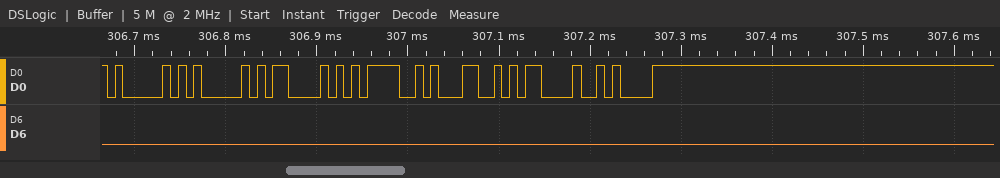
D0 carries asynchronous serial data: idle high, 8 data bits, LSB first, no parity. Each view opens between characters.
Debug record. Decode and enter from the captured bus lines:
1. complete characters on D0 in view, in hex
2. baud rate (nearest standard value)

41, 41, 43, 3D, 31, 0D, 0A
115200 baud
